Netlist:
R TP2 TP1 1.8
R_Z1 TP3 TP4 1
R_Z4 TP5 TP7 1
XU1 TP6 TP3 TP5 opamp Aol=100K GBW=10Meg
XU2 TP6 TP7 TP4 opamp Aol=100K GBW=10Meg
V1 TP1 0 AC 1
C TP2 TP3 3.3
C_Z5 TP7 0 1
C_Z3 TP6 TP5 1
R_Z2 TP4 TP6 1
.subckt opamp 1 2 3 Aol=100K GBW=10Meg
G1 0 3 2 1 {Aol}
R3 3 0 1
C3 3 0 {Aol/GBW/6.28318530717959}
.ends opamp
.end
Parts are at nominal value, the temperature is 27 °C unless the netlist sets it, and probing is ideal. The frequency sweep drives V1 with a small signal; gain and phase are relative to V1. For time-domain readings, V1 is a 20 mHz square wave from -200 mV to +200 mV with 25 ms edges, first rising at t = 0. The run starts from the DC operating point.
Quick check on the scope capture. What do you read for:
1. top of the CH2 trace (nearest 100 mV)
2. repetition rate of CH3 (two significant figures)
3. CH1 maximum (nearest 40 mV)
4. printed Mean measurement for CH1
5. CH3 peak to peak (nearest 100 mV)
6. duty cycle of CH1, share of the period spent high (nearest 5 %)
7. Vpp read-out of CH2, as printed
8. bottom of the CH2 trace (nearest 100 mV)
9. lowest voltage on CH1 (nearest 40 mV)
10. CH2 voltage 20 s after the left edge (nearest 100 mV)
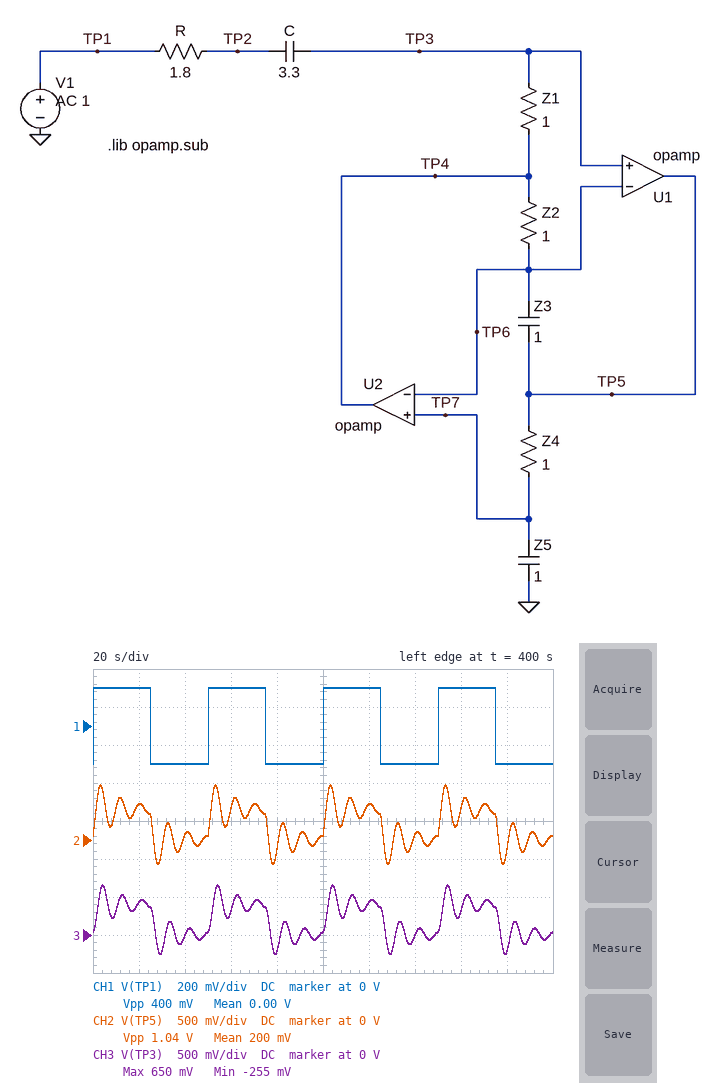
700 mV
20 mHz
200 mV
0.00 V
900 mV
50 %
1.04 V
-300 mV
-200 mV
500 mV
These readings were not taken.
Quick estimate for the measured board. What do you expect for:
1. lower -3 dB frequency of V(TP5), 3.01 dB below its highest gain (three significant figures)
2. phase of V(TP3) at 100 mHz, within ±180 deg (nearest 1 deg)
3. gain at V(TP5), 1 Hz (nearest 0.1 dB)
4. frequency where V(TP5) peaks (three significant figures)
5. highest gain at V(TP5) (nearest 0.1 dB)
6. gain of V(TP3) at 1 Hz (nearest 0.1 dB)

104 mHz
-33 deg
-20.8 dB
118 mHz
14.9 dB
-36.9 dB
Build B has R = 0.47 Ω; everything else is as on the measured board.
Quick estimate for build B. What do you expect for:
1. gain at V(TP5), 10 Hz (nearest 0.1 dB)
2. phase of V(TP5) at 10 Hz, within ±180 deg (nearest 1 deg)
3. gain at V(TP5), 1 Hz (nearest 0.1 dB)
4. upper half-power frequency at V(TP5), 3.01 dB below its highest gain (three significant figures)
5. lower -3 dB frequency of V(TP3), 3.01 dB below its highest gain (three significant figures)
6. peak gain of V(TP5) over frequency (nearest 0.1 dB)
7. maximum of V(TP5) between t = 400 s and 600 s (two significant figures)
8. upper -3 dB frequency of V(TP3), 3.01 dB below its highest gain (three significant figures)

-29.4 dB
-90 deg
-8.9 dB
282 mHz
159 mHz
12.1 dB
800 mV
268 mHz
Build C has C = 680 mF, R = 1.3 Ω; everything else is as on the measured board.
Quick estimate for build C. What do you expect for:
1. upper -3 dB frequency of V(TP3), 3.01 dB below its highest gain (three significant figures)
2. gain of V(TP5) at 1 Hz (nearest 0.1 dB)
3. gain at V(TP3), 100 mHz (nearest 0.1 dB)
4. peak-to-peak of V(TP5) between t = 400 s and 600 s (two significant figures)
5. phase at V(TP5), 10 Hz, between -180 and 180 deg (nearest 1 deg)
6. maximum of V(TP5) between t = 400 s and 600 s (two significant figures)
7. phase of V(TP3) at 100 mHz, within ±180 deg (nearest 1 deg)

150 mHz
-18.1 dB
-0.4 dB
510 mV
-90 deg
450 mV
-62 deg
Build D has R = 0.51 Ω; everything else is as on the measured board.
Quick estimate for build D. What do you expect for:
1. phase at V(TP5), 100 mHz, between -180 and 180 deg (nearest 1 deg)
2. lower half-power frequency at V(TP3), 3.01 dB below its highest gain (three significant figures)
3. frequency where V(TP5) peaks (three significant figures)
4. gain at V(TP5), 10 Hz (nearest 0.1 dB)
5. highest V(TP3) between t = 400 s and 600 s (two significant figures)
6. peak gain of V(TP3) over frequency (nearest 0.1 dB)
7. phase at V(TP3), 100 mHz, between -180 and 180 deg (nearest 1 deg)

19 deg
157 mHz
219 mHz
-30.1 dB
600 mV
7.6 dB
-13 deg
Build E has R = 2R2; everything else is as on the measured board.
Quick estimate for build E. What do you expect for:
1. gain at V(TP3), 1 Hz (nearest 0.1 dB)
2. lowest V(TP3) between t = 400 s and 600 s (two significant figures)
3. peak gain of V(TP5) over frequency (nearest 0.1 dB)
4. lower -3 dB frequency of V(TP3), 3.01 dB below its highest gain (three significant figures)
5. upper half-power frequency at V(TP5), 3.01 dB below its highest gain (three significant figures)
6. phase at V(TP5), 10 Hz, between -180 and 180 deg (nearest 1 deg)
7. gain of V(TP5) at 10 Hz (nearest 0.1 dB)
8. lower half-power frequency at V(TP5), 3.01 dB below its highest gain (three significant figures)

-38.7 dB
-320 mV
15.4 dB
94.5 mHz
117 mHz
-91 deg
-42.8 dB
95.3 mHz
